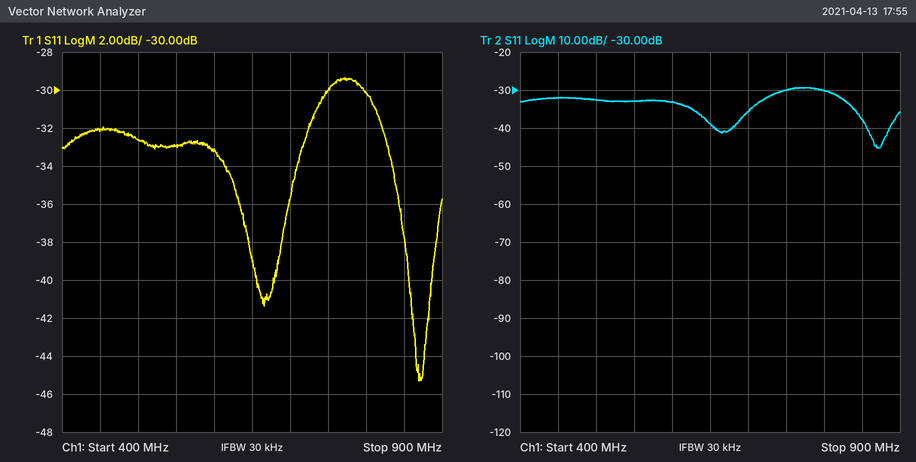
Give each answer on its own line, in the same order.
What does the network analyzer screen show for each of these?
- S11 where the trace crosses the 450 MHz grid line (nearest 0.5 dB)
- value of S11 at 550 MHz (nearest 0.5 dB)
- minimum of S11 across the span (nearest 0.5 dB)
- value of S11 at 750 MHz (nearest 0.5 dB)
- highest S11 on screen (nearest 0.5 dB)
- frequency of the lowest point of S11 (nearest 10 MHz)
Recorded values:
-32.0 dB
-33.0 dB
-45.5 dB
-30.0 dB
-29.5 dB
870 MHz
